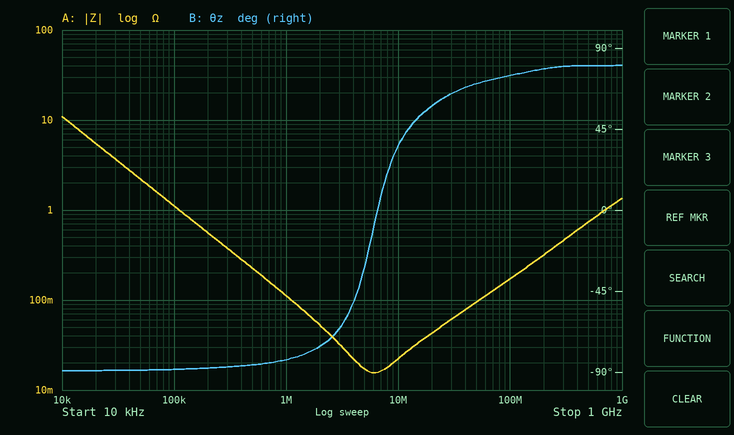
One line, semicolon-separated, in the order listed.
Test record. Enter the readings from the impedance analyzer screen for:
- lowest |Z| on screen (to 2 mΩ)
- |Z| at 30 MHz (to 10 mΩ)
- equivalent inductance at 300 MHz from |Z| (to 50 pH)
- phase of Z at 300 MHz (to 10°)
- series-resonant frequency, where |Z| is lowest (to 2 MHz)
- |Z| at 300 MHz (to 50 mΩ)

16 mΩ; 60 mΩ; 250 pH; 80°; 6 MHz; 450 mΩ
